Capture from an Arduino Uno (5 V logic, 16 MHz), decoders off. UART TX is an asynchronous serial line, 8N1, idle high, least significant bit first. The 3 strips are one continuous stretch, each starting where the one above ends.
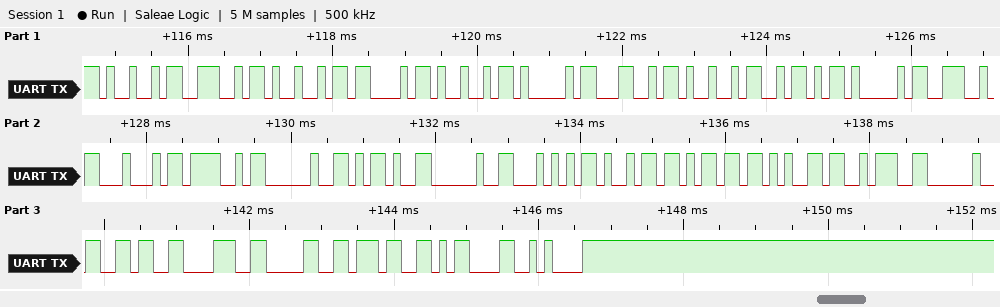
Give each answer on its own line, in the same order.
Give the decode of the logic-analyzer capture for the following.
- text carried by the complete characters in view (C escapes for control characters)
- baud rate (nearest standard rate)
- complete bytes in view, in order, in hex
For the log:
"INICIALIZANDO - Time: 6807\r\n"
9600 baud
49 4E 49 43 49 41 4C 49 5A 41 4E 44 4F 20 2D 20 54 69 6D 65 3A 20 36 38 30 37 0D 0A
